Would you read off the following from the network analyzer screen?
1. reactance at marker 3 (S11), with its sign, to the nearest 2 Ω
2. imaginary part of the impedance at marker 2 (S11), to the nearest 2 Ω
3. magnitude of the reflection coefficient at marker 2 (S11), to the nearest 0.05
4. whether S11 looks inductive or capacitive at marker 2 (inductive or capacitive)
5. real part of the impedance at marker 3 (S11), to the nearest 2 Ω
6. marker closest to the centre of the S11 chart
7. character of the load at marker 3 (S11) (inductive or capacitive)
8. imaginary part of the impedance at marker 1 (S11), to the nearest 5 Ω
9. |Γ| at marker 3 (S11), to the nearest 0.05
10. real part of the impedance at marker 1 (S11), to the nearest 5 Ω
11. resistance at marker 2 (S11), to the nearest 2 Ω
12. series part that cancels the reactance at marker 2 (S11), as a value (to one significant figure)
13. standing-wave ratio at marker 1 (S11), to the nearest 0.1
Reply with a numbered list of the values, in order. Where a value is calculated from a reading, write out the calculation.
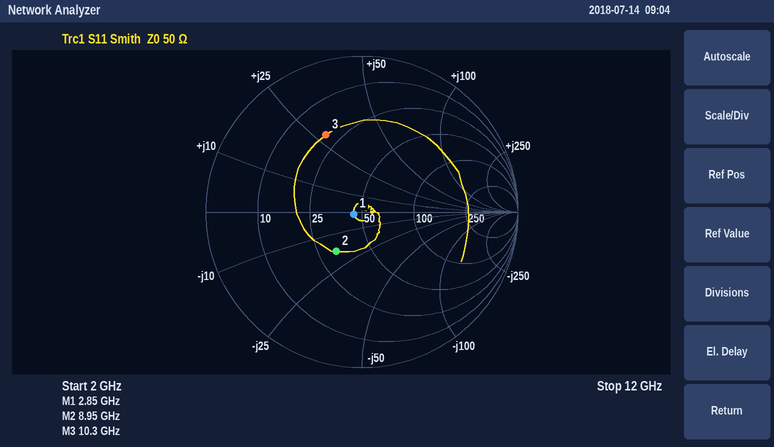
1. +28 Ω
2. -18 Ω
3. 0.30
4. capacitive
5. 20 Ω
6. marker 1
7. inductive
8. 0 Ω
9. 0.55
10. 45 Ω
11. 32 Ω
12. L = 18 Ω/(2π × 8.95 GHz) ≈ 320 pH, so 300 pH to one significant figure
13. 1.1
